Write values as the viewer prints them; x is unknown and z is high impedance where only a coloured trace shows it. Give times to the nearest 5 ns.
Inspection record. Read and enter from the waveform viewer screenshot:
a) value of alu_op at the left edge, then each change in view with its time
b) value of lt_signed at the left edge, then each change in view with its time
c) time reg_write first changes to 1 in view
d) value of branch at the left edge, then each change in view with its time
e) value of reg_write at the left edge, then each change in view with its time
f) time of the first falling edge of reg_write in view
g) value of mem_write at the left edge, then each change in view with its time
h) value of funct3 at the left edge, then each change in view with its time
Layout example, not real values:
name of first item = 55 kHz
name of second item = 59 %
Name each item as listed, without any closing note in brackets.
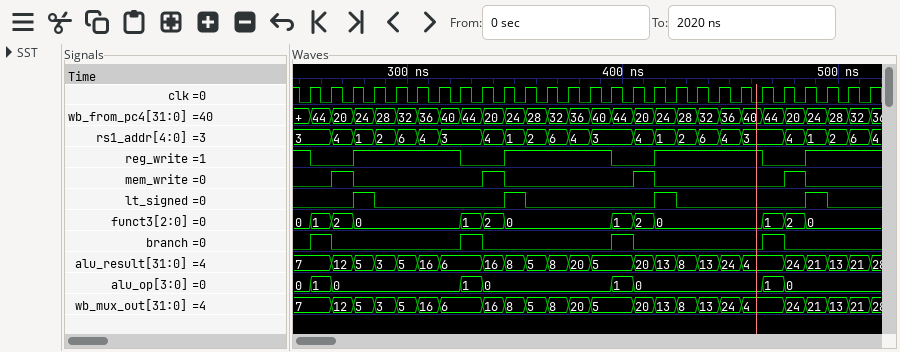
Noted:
value of alu_op at the left edge, then each change in view with its time = 0, 1 at 255 ns, 0 at 265 ns, 1 at 325 ns, 0 at 335 ns, 1 at 395 ns, 0 at 405 ns, 1 at 465 ns, 0 at 475 ns
value of lt_signed at the left edge, then each change in view with its time = 0, 1 at 275 ns, 0 at 285 ns, 1 at 345 ns, 0 at 355 ns, 1 at 415 ns, 0 at 425 ns, 1 at 485 ns, 0 at 495 ns
time reg_write first changes to 1 in view = 275 ns
value of branch at the left edge, then each change in view with its time = 0, 1 at 255 ns, 0 at 265 ns, 1 at 325 ns, 0 at 335 ns, 1 at 395 ns, 0 at 405 ns, 1 at 465 ns, 0 at 475 ns
value of reg_write at the left edge, then each change in view with its time = 1, 0 at 255 ns, 1 at 275 ns, 0 at 325 ns, 1 at 345 ns, 0 at 395 ns, 1 at 415 ns, 0 at 465 ns, 1 at 485 ns
time of the first falling edge of reg_write in view = 255 ns
value of mem_write at the left edge, then each change in view with its time = 0, 1 at 265 ns, 0 at 275 ns, 1 at 335 ns, 0 at 345 ns, 1 at 405 ns, 0 at 415 ns, 1 at 475 ns, 0 at 485 ns
value of funct3 at the left edge, then each change in view with its time = 0, 1 at 255 ns, 2 at 265 ns, 0 at 275 ns, 1 at 325 ns, 2 at 335 ns, 0 at 345 ns, 1 at 395 ns, 2 at 405 ns, 0 at 415 ns, 1 at 465 ns, 2 at 475 ns, 0 at 485 ns
